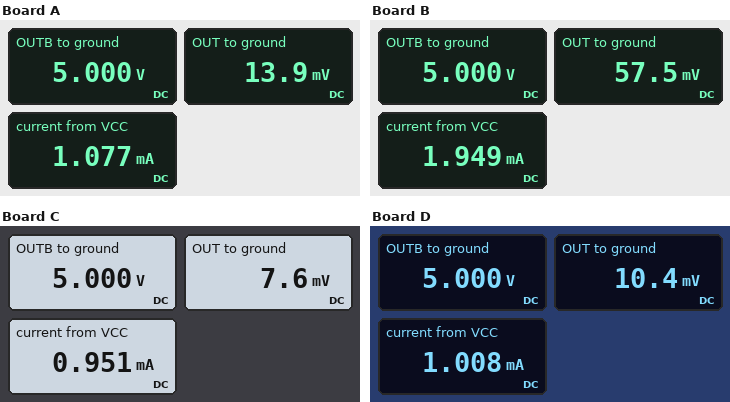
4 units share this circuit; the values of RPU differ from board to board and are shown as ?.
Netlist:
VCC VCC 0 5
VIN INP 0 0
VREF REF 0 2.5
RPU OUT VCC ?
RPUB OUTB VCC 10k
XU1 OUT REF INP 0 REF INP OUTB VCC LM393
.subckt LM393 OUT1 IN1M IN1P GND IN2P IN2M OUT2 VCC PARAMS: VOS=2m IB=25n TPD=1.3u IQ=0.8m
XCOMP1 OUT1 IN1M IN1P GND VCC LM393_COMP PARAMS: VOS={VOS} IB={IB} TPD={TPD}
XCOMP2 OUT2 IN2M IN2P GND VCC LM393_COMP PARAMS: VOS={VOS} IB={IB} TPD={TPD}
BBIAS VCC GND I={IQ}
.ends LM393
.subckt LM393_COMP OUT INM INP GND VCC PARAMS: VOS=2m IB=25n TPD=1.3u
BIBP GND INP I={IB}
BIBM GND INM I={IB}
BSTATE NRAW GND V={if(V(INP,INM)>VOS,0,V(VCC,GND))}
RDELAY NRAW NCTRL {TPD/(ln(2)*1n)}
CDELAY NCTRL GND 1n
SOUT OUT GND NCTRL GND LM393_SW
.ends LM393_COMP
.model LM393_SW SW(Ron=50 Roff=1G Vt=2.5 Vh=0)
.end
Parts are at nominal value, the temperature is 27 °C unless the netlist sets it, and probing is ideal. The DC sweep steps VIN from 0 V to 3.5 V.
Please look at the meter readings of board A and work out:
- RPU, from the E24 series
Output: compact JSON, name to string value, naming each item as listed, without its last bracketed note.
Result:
{"RPU, from the E24 series": "18 kΩ"}
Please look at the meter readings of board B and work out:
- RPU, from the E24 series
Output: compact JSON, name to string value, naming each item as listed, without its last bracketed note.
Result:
{"RPU, from the E24 series": "4.3 kΩ"}
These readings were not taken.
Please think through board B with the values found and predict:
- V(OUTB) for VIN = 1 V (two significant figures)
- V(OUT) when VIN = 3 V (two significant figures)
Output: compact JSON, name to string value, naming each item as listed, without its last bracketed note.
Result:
{"V(OUTB) for VIN = 1 V": "5.0 V", "V(OUT) when VIN = 3 V": "5.0 V"}
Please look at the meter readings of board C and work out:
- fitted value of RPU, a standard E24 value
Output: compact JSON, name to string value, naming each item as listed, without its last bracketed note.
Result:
{"fitted value of RPU, a standard E24 value": "33 kΩ"}
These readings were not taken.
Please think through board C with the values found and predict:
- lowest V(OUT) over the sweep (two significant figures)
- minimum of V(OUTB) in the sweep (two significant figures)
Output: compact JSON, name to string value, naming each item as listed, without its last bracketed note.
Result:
{"lowest V(OUT) over the sweep": "7.6 mV", "minimum of V(OUTB) in the sweep": "25 mV"}
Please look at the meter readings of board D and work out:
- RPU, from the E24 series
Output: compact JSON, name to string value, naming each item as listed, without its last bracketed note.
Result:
{"RPU, from the E24 series": "24 kΩ"}
